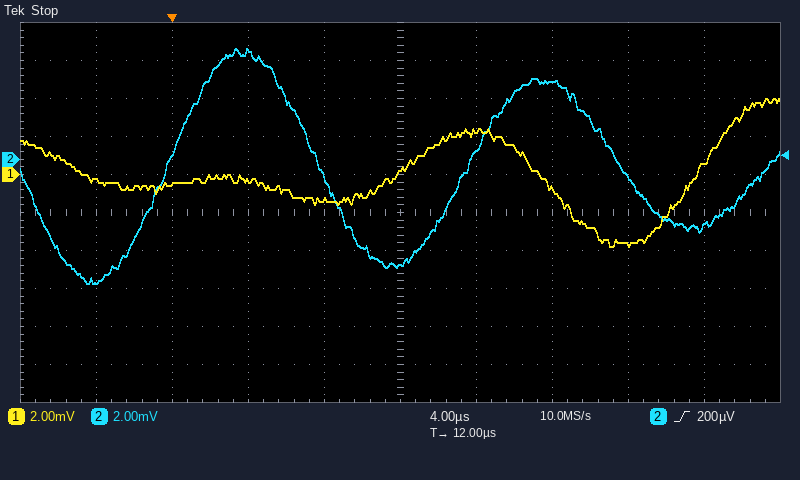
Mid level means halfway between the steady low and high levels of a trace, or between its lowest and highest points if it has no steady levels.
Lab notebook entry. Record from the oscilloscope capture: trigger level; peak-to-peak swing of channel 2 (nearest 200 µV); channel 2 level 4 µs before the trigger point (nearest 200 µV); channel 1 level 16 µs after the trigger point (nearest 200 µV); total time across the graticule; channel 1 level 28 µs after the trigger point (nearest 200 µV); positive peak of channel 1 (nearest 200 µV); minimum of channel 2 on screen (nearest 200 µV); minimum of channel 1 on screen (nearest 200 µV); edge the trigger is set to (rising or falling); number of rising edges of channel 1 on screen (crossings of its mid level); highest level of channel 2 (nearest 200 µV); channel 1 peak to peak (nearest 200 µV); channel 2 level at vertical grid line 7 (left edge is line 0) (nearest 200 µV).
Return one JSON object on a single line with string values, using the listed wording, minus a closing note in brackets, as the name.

{"trigger level": "200 µV", "peak-to-peak swing of channel 2": "12.4 mV", "channel 2 level 4 µs before the trigger point": "-6.4 mV", "channel 1 level 16 µs after the trigger point": "2.2 mV", "total time across the graticule": "40 µs", "channel 1 level 28 µs after the trigger point": "600 µV", "positive peak of channel 1": "4.0 mV", "minimum of channel 2 on screen": "-6.6 mV", "minimum of channel 1 on screen": "-3.8 mV", "edge the trigger is set to": "rising", "number of rising edges of channel 1 on screen": "2", "highest level of channel 2": "5.8 mV", "channel 1 peak to peak": "7.8 mV", "channel 2 level at vertical grid line 7 (left edge is line 0)": "4.0 mV"}
